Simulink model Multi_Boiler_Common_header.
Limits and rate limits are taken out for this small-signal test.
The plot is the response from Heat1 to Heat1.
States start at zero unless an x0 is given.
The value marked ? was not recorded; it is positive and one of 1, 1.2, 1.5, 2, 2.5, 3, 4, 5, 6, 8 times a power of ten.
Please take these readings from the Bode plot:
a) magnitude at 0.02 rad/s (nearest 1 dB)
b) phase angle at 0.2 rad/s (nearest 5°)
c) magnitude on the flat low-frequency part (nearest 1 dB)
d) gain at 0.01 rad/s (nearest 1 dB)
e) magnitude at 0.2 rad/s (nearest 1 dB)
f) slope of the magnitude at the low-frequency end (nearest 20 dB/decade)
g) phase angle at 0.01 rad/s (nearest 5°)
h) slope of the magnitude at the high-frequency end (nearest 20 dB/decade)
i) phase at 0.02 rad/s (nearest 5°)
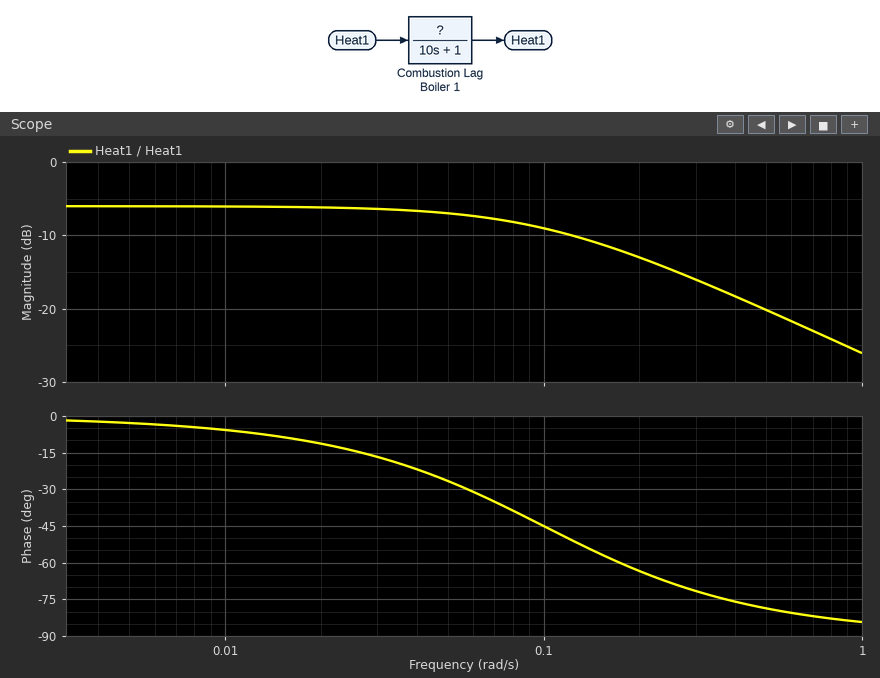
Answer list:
-6 dB
-65°
-6 dB
-6 dB
-13 dB
0 dB/decade
-5°
-20 dB/decade
-10°
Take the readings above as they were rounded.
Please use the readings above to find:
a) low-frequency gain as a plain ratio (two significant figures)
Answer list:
0.50
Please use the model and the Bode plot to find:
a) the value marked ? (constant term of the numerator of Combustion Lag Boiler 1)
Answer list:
0.5
